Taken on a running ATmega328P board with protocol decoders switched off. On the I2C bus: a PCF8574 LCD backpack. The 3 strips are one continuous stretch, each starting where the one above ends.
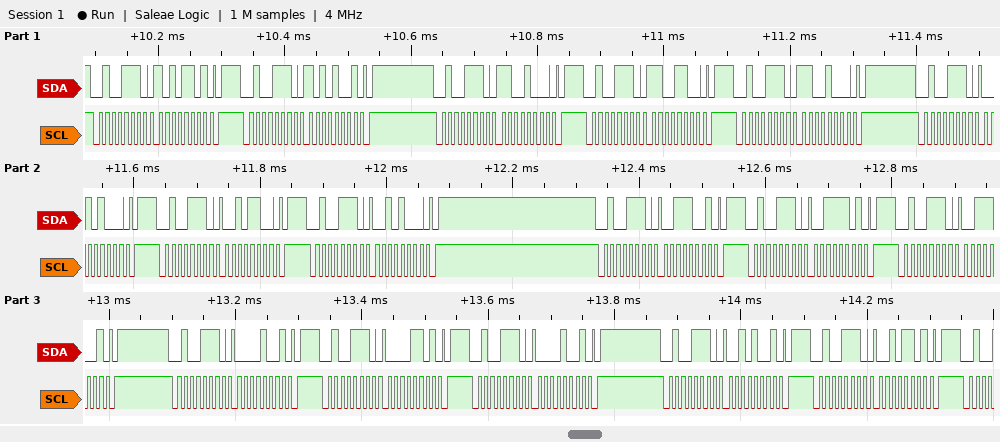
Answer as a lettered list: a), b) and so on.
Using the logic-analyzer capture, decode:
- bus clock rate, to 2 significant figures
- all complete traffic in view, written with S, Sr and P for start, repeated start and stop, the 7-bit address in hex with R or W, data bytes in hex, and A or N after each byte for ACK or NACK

a) 100 kHz
b) S 27W A AD A P S 27W A A9 A P S 27W A C8 A P S 27W A CC A P S 27W A C8 A P S 27W A 28 A P S 27W A 2C A P S 27W A 28 A P S 27W A 39 A P S 27W A 3D A P S 27W A 39 A P S 27W A 09 A P S 27W A 0D A P S 27W A 09 A P S 27W A 29 A P S 27W A 2D A P
